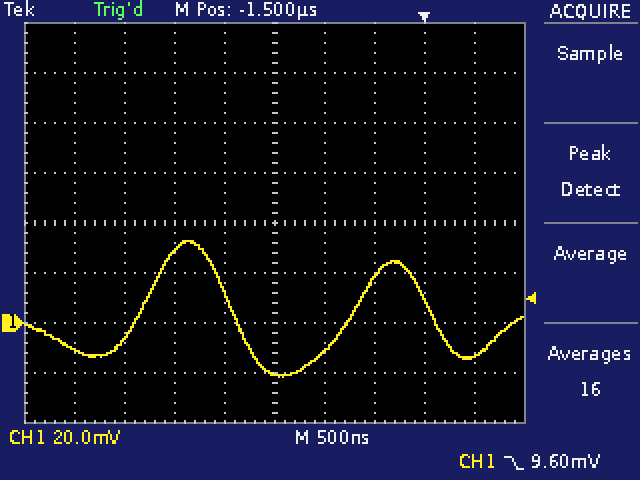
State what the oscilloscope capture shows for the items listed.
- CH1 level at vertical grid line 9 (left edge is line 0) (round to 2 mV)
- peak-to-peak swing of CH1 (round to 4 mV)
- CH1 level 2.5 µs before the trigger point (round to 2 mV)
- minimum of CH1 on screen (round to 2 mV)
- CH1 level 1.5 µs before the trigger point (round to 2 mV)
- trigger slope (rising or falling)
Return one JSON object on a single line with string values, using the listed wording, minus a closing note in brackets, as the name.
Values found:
{"CH1 level at vertical grid line 9 (left edge is line 0)": "-14 mV", "peak-to-peak swing of CH1": "56 mV", "CH1 level 2.5 µs before the trigger point": "28 mV", "minimum of CH1 on screen": "-22 mV", "CH1 level 1.5 µs before the trigger point": "-20 mV", "trigger slope": "falling"}
